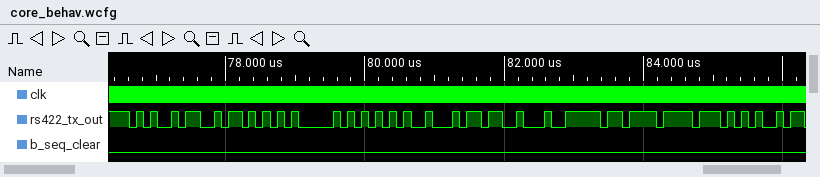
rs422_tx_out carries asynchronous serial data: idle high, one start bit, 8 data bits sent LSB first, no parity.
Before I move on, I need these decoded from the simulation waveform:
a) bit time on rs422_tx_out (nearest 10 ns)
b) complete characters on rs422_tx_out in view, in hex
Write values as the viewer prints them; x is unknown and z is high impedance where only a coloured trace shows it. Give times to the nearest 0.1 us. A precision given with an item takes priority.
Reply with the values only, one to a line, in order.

100 ns
A5, 5A, 05, 55, A2, 13, BE, EF, 57
